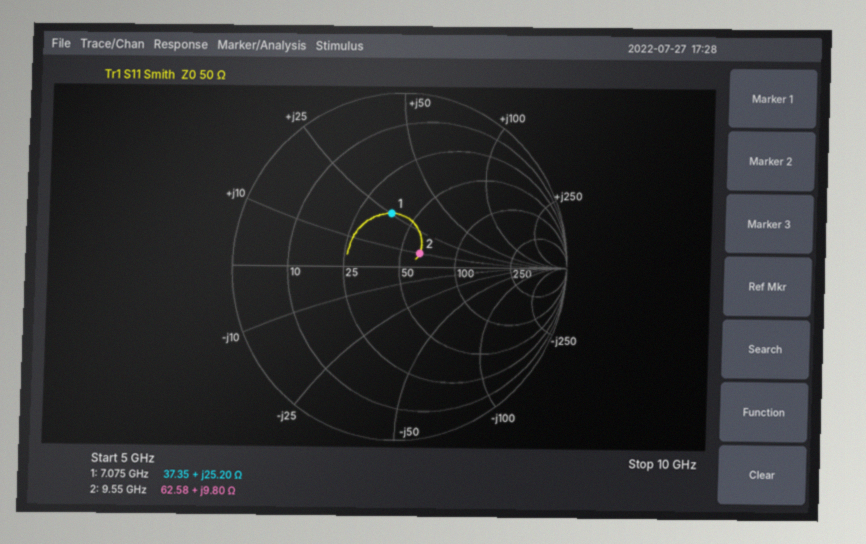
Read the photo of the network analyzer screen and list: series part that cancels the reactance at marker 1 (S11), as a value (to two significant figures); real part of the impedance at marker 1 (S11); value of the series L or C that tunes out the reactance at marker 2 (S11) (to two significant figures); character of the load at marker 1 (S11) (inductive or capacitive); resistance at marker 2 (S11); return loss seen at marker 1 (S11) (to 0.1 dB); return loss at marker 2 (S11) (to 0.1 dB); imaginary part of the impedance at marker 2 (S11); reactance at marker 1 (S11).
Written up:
890 fF
37.35 Ω
1.7 pF
inductive
62.58 Ω
10.2 dB
17.0 dB
+9.80 Ω
+25.20 Ω
